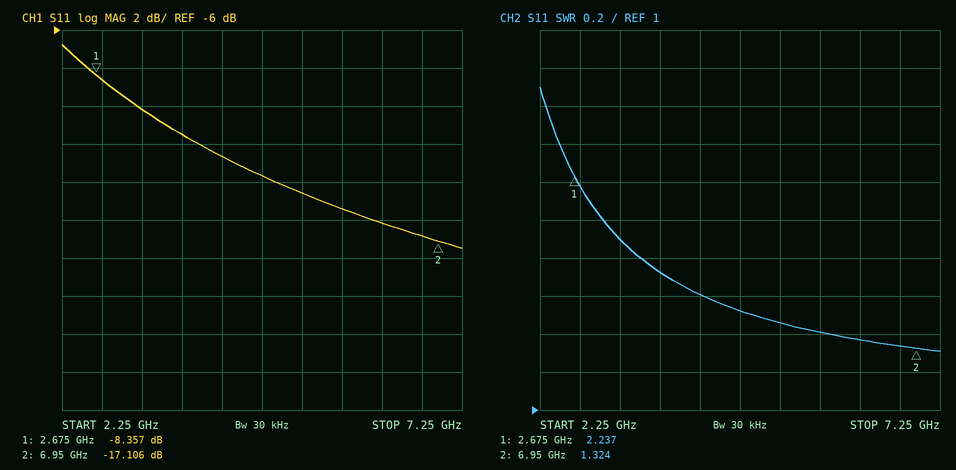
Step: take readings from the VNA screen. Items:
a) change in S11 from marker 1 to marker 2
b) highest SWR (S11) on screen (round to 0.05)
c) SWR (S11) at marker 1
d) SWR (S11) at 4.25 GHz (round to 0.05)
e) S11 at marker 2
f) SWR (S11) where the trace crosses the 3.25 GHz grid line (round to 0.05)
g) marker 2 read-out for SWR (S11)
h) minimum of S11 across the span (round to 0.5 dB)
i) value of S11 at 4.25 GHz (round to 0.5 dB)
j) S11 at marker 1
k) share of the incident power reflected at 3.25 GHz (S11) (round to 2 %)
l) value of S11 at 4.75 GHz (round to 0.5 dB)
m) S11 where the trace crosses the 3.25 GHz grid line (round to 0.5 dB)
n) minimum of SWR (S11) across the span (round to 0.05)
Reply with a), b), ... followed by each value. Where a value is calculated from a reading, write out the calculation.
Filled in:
a) -17.106 − (-8.357) = -8.749 dB
b) 2.70
c) 2.237
d) 1.60
e) -17.106 dB
f) 1.90
g) 1.324
h) -17.5 dB
i) -12.5 dB
j) -8.357 dB
k) 10^(-10/10) ≈ 10 %
l) -13.5 dB
m) -10.0 dB
n) 1.30
